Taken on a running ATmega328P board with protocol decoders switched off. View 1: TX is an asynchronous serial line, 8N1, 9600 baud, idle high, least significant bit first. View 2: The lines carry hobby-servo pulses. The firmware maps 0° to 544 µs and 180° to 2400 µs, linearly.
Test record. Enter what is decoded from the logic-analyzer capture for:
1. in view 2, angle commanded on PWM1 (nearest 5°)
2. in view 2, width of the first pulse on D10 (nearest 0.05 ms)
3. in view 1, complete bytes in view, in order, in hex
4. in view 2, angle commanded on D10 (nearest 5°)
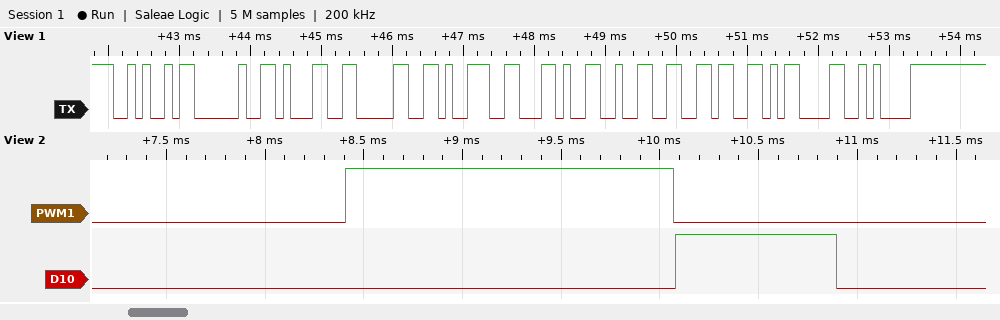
110°
0.80 ms
0x4A 0x20 0x31 0x30 0x39 0x2C 0x32 0x36 0x0D 0x0A
25°
